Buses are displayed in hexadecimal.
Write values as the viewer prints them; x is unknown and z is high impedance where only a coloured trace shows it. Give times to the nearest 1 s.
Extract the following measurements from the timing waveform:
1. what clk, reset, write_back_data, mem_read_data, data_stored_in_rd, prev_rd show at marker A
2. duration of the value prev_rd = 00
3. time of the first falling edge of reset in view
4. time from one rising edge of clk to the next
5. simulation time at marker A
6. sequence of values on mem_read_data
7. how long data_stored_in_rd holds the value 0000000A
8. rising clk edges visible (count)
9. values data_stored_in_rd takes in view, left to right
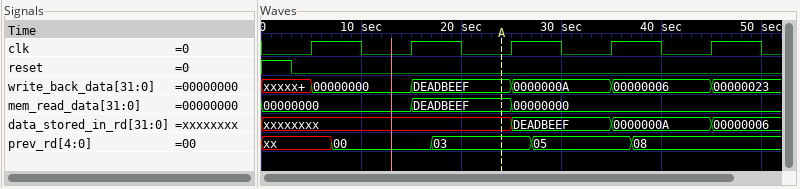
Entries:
clk=0, reset=0, write_back_data=DEADBEEF, mem_read_data=DEADBEEF, data_stored_in_rd=xxxxxxxx, prev_rd=03
10 s
3 s
10 s
24 s
00000000, DEADBEEF, 00000000
10 s
5
xxxxxxxx, DEADBEEF, 0000000A, 00000006
